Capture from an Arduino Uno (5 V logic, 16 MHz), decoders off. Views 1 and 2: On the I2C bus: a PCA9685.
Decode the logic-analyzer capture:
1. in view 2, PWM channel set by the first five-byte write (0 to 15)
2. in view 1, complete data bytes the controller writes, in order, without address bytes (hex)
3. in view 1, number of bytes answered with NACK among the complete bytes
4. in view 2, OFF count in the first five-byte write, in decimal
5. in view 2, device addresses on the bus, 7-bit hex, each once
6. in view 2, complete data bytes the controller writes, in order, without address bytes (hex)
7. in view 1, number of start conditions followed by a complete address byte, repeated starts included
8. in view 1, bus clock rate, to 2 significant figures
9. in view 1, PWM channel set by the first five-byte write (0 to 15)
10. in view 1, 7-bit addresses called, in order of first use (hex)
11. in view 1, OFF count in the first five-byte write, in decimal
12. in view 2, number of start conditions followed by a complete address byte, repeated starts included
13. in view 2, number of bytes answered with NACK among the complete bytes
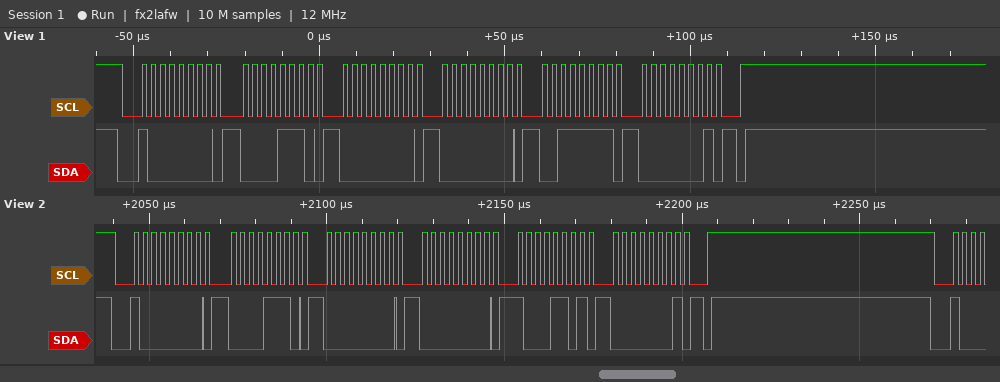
2
0E 00 00 3F 01
0
397
0x40
0E 00 00 8D 01
1
400 kHz
2
0x40
319
1
0
